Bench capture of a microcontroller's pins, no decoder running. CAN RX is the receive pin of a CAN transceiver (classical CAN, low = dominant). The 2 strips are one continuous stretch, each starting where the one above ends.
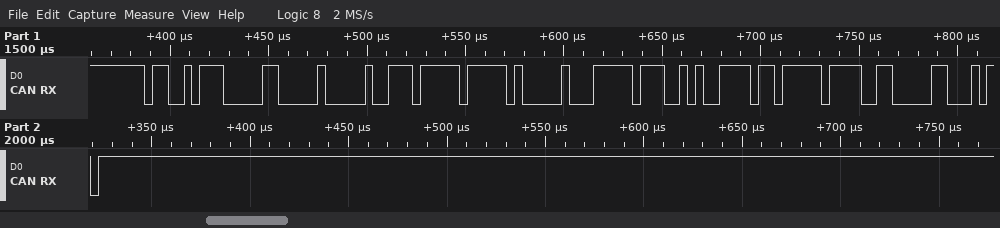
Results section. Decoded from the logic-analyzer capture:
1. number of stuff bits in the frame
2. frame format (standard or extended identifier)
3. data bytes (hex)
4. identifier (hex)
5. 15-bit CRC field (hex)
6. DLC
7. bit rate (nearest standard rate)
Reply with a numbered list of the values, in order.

1. 9
2. standard
3. 00 77 FF 00 FF 29 ED FF
4. 0x65C
5. 0x1822
6. 8
7. 250 kbit/s
